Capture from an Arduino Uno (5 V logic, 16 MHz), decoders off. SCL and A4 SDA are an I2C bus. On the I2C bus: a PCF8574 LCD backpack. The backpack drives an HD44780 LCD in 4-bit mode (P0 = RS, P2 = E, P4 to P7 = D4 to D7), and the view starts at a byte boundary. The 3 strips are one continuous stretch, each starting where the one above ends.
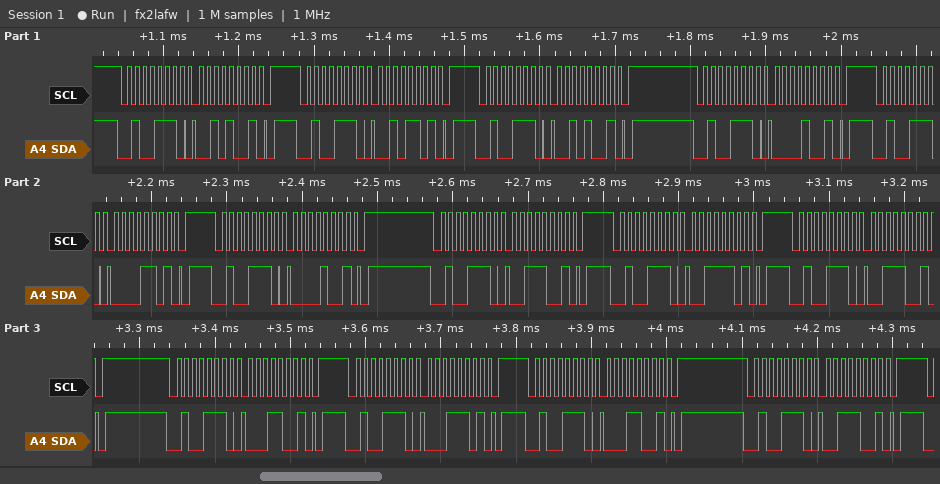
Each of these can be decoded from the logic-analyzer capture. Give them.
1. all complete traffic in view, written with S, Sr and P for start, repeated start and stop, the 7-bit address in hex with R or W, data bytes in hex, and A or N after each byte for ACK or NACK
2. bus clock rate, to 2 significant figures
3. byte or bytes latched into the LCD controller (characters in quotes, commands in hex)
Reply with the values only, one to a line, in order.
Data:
S 27W A 29 A P S 27W A 2D A P S 27W A 29 A P S 27W A 09 A P S 27W A 0D A P S 27W A 09 A P S 27W A 39 A P S 27W A 3D A P S 27W A 39 A P S 27W A 19 A P S 27W A 1D A P S 27W A 19 A P S 27W A 39 A P
100 kHz
' ' '1'
